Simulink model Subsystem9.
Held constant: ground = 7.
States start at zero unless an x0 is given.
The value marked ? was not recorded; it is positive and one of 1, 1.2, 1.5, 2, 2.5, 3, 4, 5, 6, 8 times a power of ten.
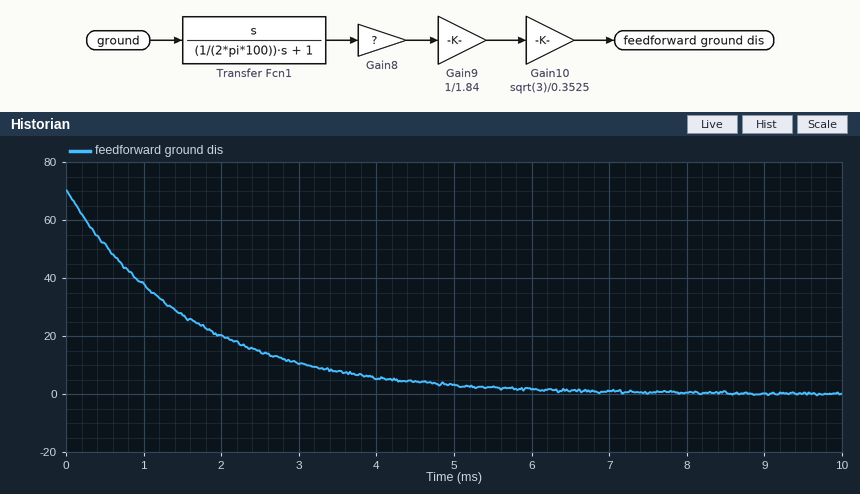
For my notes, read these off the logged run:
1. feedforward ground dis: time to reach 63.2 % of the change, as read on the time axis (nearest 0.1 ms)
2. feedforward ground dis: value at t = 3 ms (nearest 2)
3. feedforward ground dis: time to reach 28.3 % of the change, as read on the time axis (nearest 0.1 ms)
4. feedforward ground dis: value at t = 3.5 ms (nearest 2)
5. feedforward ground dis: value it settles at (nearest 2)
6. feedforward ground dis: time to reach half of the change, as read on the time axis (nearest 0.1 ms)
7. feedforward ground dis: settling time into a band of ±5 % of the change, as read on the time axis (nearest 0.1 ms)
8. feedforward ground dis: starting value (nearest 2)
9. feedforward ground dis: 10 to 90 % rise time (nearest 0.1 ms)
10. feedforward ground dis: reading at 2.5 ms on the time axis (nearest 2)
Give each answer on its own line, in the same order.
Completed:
1.6 ms
10
0.5 ms
8
0
1.1 ms
4.8 ms
70
3.5 ms
14
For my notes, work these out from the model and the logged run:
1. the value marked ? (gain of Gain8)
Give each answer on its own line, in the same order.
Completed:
0.006
